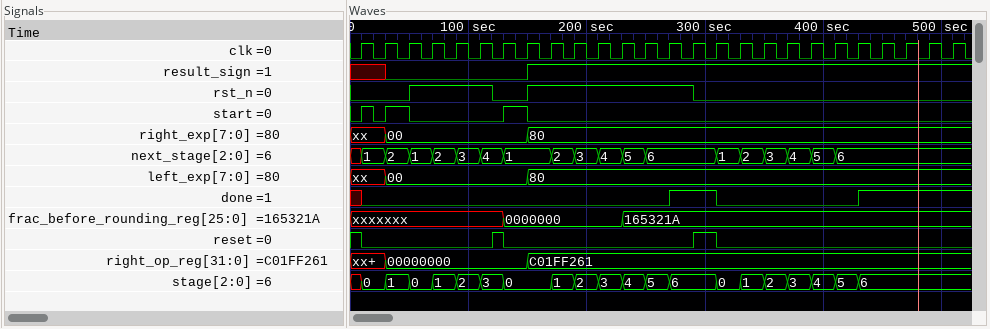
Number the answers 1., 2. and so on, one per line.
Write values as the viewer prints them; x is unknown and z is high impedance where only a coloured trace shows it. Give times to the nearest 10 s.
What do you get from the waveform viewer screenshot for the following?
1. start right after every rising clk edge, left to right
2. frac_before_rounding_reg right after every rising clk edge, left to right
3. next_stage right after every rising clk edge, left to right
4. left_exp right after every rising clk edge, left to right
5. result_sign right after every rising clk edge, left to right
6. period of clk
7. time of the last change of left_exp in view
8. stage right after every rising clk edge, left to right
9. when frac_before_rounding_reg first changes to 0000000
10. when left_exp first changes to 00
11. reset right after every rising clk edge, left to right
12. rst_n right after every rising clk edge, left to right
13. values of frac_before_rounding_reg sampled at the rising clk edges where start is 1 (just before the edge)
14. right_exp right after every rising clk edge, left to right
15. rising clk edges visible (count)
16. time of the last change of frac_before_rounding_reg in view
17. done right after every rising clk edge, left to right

1. 1 1 0 0 0 0 1 0 0 0 0 0 0 0 0 0 0 0 0 0 0 0 0 0 0 0
2. xxxxxxx, xxxxxxx, xxxxxxx, xxxxxxx, xxxxxxx, xxxxxxx, 0000000, 0000000, 0000000, 0000000, 0000000, 165321A, 165321A, 165321A, 165321A, 165321A, 165321A, 165321A, 165321A, 165321A, 165321A, 165321A, 165321A, 165321A, 165321A, 165321A
3. 1, 2, 1, 2, 3, 4, 1, 1, 2, 3, 4, 5, 6, 6, 6, 1, 2, 3, 4, 5, 6, 6, 6, 6, 6, 6
4. xx, 00, 00, 00, 00, 00, 00, 80, 80, 80, 80, 80, 80, 80, 80, 80, 80, 80, 80, 80, 80, 80, 80, 80, 80, 80
5. x 0 0 0 0 0 0 1 1 1 1 1 1 1 1 1 1 1 1 1 1 1 1 1 1 1
6. 20 s
7. 150 s
8. 0, 1, 0, 1, 2, 3, 0, 0, 1, 2, 3, 4, 5, 6, 6, 0, 1, 2, 3, 4, 5, 6, 6, 6, 6, 6
9. 130 s
10. 30 s
11. 0 0 0 0 0 0 0 0 0 0 0 0 0 0 1 0 0 0 0 0 0 0 0 0 0 0
12. 0 0 1 1 1 1 0 1 1 1 1 1 1 1 0 0 0 0 0 0 0 0 0 0 0 0
13. xxxxxxx, 0000000
14. xx, 00, 00, 00, 00, 00, 00, 80, 80, 80, 80, 80, 80, 80, 80, 80, 80, 80, 80, 80, 80, 80, 80, 80, 80, 80
15. 26
16. 230 s
17. 0 0 0 0 0 0 0 0 0 0 0 0 0 1 1 0 0 0 0 0 0 1 1 1 1 1
